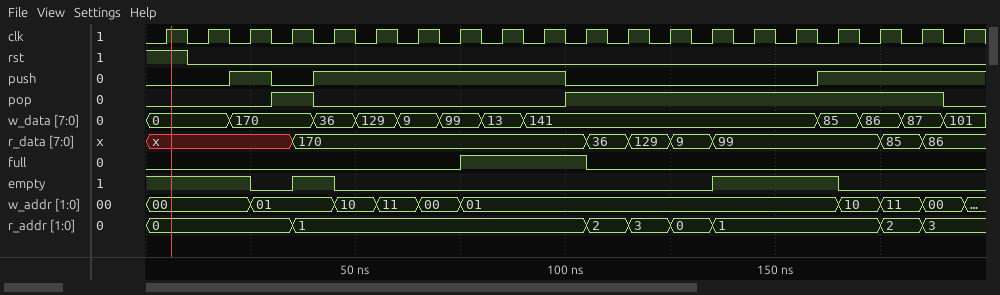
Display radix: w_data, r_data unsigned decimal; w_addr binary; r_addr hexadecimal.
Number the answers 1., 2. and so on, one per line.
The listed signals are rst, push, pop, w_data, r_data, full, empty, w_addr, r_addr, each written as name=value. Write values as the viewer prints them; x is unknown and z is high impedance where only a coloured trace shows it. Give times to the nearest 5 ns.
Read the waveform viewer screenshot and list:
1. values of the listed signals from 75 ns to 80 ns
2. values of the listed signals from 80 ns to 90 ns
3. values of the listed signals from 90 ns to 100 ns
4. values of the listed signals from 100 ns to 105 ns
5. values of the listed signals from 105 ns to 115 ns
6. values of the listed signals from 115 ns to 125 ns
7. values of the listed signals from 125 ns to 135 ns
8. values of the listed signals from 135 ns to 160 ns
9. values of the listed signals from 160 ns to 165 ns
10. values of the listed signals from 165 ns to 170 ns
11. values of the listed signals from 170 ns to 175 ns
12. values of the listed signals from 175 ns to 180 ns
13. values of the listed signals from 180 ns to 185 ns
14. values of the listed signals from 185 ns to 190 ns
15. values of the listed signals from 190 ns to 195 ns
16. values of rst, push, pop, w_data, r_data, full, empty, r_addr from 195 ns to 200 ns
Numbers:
1. rst=0, push=1, pop=0, w_data=99, r_data=170, full=1, empty=0, w_addr=01, r_addr=1
2. rst=0, push=1, pop=0, w_data=13, r_data=170, full=1, empty=0, w_addr=01, r_addr=1
3. rst=0, push=1, pop=0, w_data=141, r_data=170, full=1, empty=0, w_addr=01, r_addr=1
4. rst=0, push=0, pop=1, w_data=141, r_data=170, full=1, empty=0, w_addr=01, r_addr=1
5. rst=0, push=0, pop=1, w_data=141, r_data=36, full=0, empty=0, w_addr=01, r_addr=2
6. rst=0, push=0, pop=1, w_data=141, r_data=129, full=0, empty=0, w_addr=01, r_addr=3
7. rst=0, push=0, pop=1, w_data=141, r_data=9, full=0, empty=0, w_addr=01, r_addr=0
8. rst=0, push=0, pop=1, w_data=141, r_data=99, full=0, empty=1, w_addr=01, r_addr=1
9. rst=0, push=1, pop=1, w_data=85, r_data=99, full=0, empty=1, w_addr=01, r_addr=1
10. rst=0, push=1, pop=1, w_data=85, r_data=99, full=0, empty=0, w_addr=10, r_addr=1
11. rst=0, push=1, pop=1, w_data=86, r_data=99, full=0, empty=0, w_addr=10, r_addr=1
12. rst=0, push=1, pop=1, w_data=86, r_data=85, full=0, empty=0, w_addr=11, r_addr=2
13. rst=0, push=1, pop=1, w_data=87, r_data=85, full=0, empty=0, w_addr=11, r_addr=2
14. rst=0, push=1, pop=1, w_data=87, r_data=86, full=0, empty=0, w_addr=00, r_addr=3
15. rst=0, push=1, pop=0, w_data=101, r_data=86, full=0, empty=0, w_addr=00, r_addr=3
16. rst=0, push=1, pop=0, w_data=101, r_data=86, full=0, empty=0, r_addr=3
